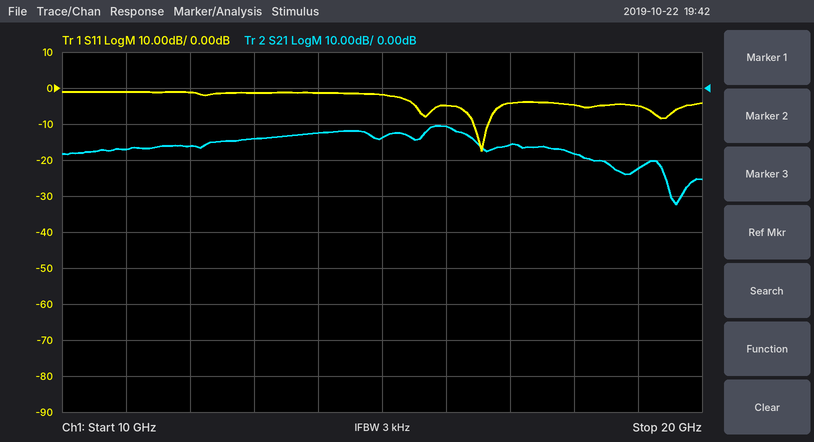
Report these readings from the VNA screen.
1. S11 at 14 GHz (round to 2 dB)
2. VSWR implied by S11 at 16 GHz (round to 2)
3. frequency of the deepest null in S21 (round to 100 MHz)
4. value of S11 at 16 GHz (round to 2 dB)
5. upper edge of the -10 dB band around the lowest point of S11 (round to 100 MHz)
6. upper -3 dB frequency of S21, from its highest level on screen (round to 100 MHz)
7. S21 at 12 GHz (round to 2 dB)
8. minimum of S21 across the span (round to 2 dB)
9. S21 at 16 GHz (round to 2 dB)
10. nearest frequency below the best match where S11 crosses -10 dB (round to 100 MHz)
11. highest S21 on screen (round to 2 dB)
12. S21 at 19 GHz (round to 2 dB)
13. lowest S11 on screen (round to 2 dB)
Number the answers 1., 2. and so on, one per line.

1. -2 dB
2. 4
3. 19.6 GHz
4. -4 dB
5. 16.7 GHz
6. 16.4 GHz
7. -16 dB
8. -32 dB
9. -10 dB
10. 16.4 GHz
11. -10 dB
12. -22 dB
13. -18 dB
